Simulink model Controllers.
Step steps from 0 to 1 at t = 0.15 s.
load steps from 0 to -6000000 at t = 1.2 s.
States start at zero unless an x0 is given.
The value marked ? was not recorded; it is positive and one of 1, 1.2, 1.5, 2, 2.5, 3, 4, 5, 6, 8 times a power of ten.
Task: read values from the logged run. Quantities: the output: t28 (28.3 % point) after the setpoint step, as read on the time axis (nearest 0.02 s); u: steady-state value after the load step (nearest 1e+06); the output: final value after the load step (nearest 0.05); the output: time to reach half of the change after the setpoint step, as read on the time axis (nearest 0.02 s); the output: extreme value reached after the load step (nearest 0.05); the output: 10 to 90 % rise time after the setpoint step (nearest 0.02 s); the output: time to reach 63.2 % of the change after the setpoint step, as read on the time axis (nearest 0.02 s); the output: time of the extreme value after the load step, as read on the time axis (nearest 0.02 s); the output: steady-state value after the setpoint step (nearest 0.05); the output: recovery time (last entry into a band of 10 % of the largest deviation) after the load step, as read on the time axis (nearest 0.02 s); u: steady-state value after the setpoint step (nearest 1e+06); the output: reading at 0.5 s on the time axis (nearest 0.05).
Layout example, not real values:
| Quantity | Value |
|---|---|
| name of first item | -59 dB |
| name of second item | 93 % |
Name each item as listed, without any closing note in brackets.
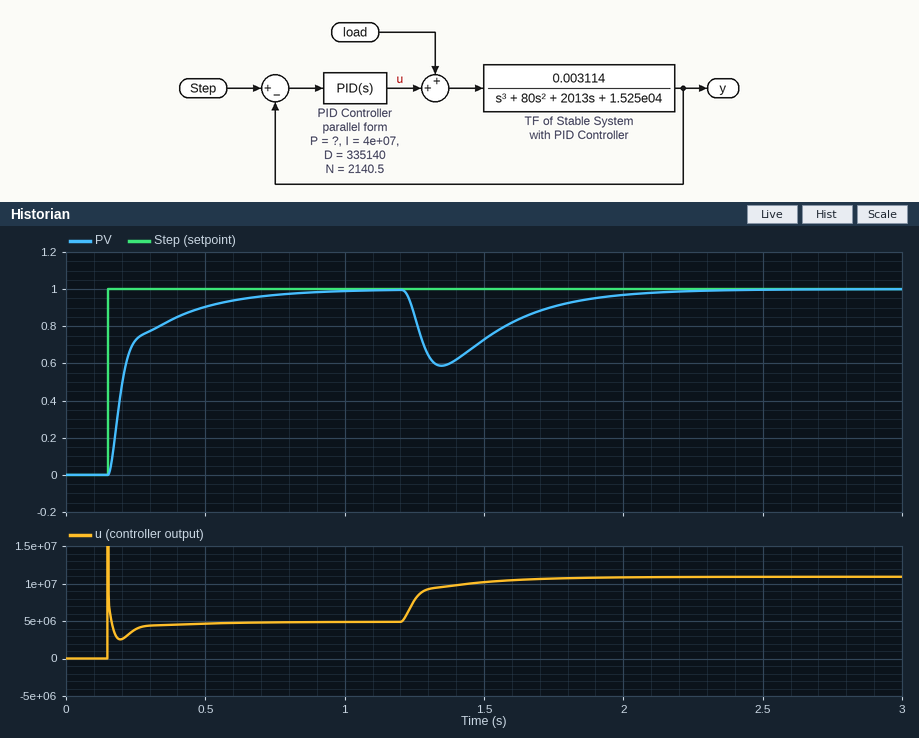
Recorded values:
| Quantity | Value |
|---|---|
| the output: t28 (28.3 % point) after the setpoint step, as read on the time axis | 0.18 s |
| u: steady-state value after the load step | 11000000 |
| the output: final value after the load step | 1.00 |
| the output: time to reach half of the change after the setpoint step, as read on the time axis | 0.20 s |
| the output: extreme value reached after the load step | 0.60 |
| the output: 10 to 90 % rise time after the setpoint step | 0.32 s |
| the output: time to reach 63.2 % of the change after the setpoint step, as read on the time axis | 0.22 s |
| the output: time of the extreme value after the load step, as read on the time axis | 1.34 s |
| the output: steady-state value after the setpoint step | 1.00 |
| the output: recovery time (last entry into a band of 10 % of the largest deviation) after the load step, as read on the time axis | 1.94 s |
| u: steady-state value after the setpoint step | 5000000 |
| the output: reading at 0.5 s on the time axis | 0.90 |
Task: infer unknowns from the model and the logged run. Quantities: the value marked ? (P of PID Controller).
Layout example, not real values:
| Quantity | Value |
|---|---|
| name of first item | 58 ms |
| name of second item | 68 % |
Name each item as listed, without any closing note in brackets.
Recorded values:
| Quantity | Value |
|---|---|
| the value marked ? | 8e+06 |
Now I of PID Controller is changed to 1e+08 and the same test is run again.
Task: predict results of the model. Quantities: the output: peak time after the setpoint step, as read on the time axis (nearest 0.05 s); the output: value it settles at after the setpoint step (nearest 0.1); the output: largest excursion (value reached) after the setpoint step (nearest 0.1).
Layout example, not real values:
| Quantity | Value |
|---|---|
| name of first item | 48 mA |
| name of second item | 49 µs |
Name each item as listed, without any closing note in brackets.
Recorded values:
| Quantity | Value |
|---|---|
| the output: peak time after the setpoint step, as read on the time axis | 0.40 s |
| the output: value it settles at after the setpoint step | 1.0 |
| the output: largest excursion (value reached) after the setpoint step | 1.1 |
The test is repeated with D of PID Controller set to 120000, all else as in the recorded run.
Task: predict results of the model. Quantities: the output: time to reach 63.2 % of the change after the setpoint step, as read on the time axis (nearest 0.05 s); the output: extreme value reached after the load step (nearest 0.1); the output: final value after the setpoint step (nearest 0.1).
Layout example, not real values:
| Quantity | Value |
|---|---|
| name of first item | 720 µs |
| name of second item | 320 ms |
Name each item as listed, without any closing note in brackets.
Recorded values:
| Quantity | Value |
|---|---|
| the output: time to reach 63.2 % of the change after the setpoint step, as read on the time axis | 0.25 s |
| the output: extreme value reached after the load step | 0.5 |
| the output: final value after the setpoint step | 1.0 |
